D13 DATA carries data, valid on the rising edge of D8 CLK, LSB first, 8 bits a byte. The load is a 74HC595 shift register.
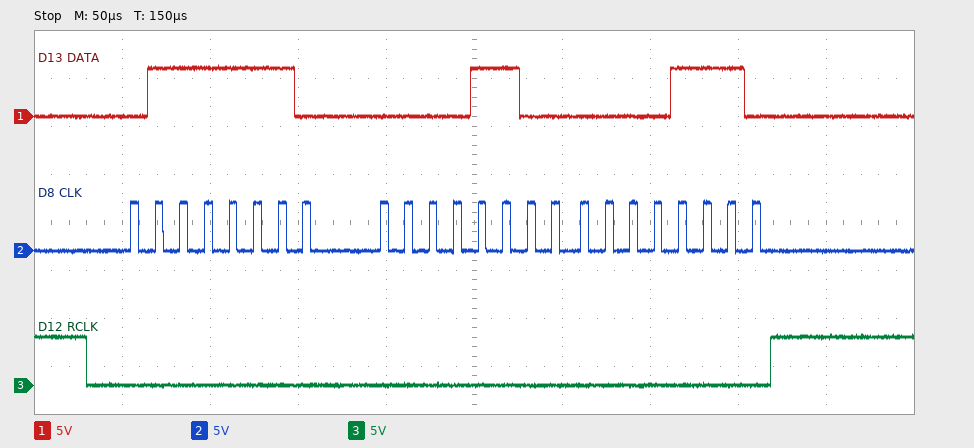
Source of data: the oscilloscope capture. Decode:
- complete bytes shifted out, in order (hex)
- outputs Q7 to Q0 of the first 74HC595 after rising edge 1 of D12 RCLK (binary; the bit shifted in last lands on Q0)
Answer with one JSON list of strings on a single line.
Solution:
["0x7E 0x30 0x70", "00001110"]
